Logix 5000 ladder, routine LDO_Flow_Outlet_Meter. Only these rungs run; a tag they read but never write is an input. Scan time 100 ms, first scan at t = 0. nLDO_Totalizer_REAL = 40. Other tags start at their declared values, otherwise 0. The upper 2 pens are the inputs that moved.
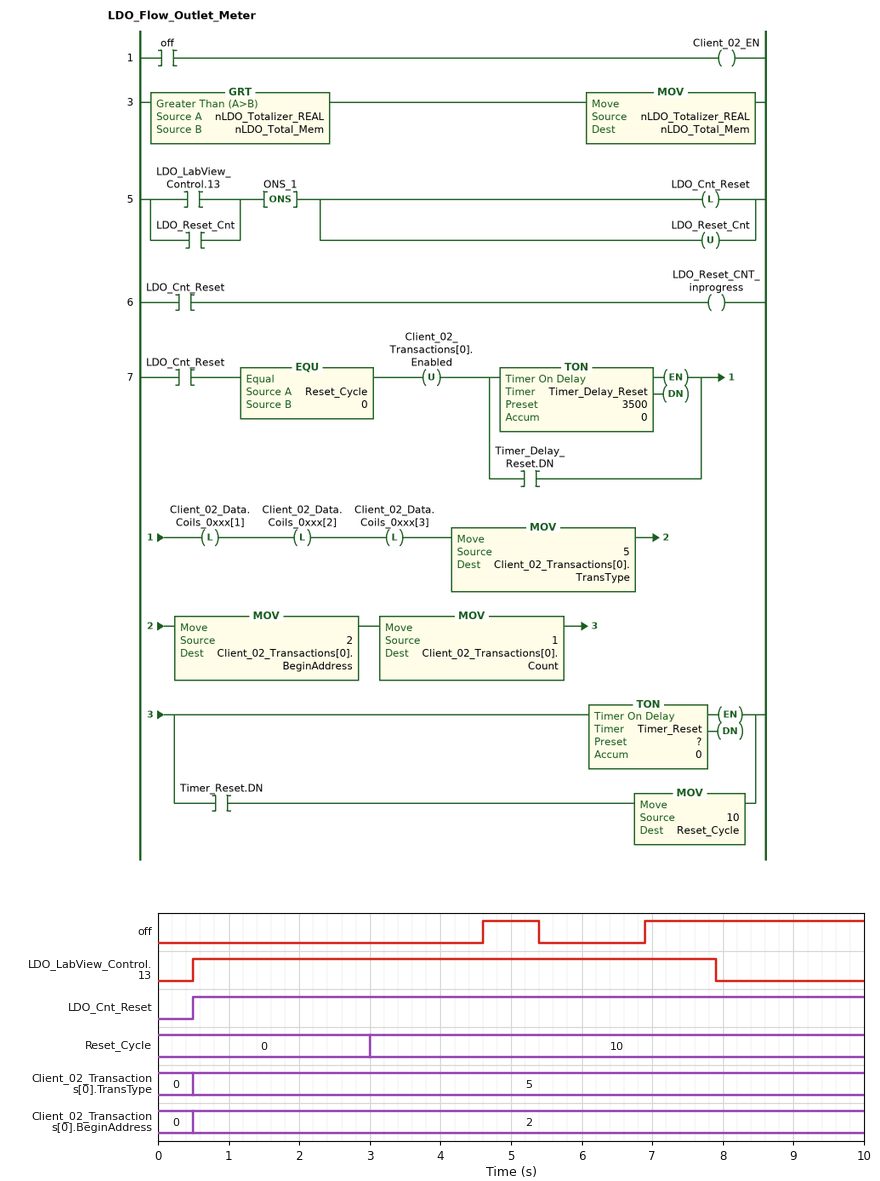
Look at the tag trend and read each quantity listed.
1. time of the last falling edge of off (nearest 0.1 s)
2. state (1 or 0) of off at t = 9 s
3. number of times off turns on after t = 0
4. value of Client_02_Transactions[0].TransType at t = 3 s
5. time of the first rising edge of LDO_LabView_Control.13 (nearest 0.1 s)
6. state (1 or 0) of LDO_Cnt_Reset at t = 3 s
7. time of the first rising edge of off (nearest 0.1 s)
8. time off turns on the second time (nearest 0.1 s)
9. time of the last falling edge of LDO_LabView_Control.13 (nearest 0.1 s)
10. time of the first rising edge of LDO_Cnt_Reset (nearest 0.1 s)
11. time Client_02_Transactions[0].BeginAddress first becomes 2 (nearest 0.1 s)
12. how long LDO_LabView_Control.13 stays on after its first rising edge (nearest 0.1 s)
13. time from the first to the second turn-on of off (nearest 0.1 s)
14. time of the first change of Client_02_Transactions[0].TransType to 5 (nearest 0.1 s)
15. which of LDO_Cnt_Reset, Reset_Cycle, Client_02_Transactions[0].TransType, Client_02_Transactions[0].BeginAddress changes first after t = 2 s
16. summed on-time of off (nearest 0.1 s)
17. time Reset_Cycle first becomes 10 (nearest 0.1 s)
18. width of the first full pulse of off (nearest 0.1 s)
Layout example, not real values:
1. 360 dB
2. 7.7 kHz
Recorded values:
1. 5.4 s
2. 1
3. 2
4. 5
5. 0.5 s
6. 1
7. 4.6 s
8. 6.9 s
9. 7.9 s
10. 0.5 s
11. 0.5 s
12. 7.4 s
13. 2.3 s
14. 0.5 s
15. Reset_Cycle
16. 3.9 s
17. 3.0 s
18. 0.8 s
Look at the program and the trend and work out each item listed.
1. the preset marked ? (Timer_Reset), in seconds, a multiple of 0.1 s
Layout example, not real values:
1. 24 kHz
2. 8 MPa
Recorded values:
1. 2.5 s
